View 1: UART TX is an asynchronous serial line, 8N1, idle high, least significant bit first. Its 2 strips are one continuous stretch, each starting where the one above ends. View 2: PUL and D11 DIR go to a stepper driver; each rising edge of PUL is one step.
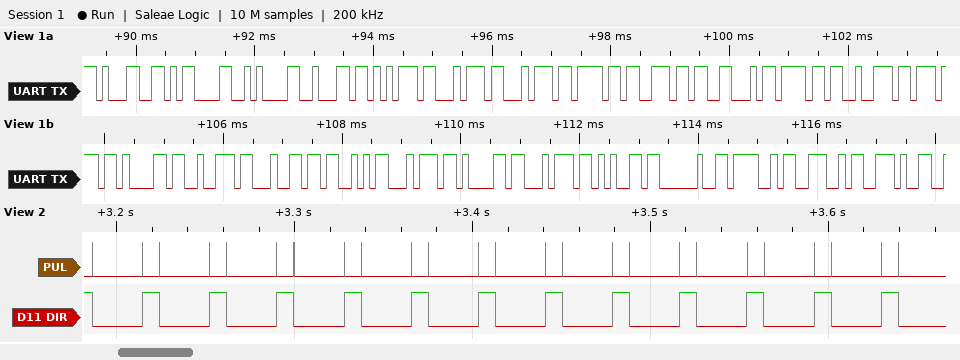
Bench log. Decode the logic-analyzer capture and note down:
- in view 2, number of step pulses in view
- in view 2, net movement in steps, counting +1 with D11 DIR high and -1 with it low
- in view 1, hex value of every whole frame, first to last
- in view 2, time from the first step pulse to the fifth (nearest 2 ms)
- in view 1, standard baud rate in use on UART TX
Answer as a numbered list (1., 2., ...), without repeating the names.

1. 25
2. -1
3. 0x31 0x0D 0x0A 0x62 0x75 0x74 0x74 0x6F 0x6E 0x46 0x6F 0x72 0x77 0x61 0x72 0x64 0x53 0x74 0x61 0x74 0x65 0x20 0x4F 0x4E 0x2E
4. 76 ms
5. 9600 baud
